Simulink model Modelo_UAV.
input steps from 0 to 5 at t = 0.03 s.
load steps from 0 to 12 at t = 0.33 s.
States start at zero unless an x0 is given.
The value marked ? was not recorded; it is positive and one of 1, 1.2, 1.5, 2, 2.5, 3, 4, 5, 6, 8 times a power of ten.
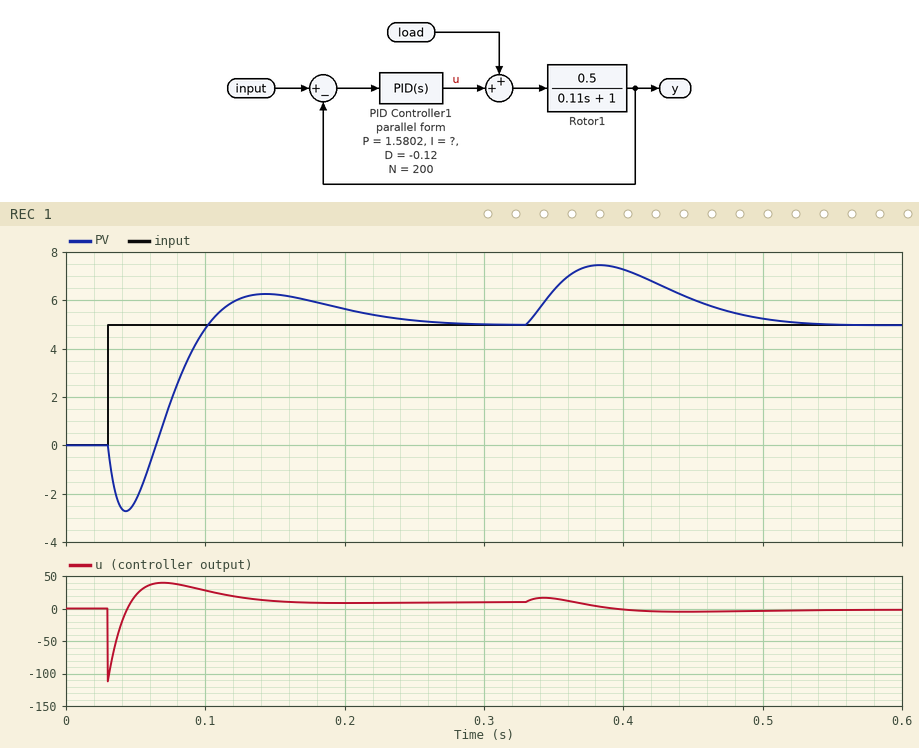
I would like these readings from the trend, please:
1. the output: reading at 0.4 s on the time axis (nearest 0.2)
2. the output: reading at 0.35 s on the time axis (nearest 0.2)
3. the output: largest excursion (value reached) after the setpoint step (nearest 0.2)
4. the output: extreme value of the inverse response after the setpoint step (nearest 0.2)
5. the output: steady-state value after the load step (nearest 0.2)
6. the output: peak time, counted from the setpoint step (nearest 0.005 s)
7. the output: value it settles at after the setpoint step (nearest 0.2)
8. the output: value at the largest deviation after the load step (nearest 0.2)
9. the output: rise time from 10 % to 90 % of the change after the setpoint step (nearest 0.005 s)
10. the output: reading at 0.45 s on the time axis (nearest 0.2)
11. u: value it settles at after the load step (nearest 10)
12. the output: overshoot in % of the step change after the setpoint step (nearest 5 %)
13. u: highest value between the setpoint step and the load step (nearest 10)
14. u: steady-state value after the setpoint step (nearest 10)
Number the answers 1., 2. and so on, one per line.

1. 7.2
2. 6.4
3. 6.2
4. -2.8
5. 5.0
6. 0.115 s
7. 5.0
8. 7.4
9. 0.030 s
10. 6.0
11. 0
12. 25 %
13. 40
14. 10
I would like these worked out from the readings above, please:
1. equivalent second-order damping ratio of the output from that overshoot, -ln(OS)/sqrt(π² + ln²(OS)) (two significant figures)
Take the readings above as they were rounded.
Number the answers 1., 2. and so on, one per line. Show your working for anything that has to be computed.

1. ln(0.25) = -1.386; 1.386 / sqrt(9.870 + 1.922) = 0.40
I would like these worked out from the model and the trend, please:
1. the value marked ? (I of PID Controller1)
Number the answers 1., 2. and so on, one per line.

1. 50
